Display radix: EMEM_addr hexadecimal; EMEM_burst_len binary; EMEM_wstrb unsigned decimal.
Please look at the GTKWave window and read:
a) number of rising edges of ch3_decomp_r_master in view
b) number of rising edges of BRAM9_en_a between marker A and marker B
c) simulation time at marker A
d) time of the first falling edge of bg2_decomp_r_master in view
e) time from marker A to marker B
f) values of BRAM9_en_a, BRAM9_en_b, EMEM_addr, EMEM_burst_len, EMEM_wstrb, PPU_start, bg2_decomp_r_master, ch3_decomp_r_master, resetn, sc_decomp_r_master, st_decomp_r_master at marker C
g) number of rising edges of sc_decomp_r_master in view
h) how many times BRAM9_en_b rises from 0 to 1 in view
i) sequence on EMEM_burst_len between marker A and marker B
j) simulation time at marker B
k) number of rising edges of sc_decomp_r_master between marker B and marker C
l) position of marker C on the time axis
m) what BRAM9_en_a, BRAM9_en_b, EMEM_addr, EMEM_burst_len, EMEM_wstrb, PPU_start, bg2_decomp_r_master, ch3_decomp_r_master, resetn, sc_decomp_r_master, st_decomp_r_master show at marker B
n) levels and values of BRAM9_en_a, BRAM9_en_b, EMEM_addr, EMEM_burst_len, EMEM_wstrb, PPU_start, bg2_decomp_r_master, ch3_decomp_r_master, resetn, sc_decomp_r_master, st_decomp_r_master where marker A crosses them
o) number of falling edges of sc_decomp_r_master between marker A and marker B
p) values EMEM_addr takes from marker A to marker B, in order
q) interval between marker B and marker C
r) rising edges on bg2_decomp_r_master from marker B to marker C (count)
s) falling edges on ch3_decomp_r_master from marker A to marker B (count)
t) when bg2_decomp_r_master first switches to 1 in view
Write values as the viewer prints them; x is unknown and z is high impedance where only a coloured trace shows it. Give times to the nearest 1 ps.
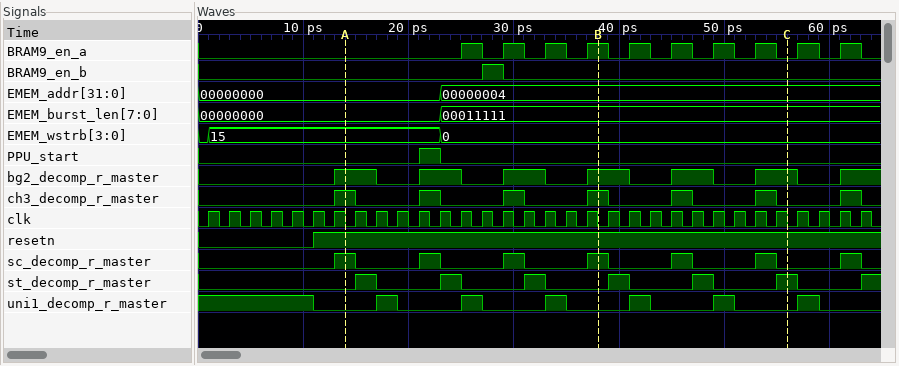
7
4
14 ps
17 ps
24 ps
BRAM9_en_a=0, BRAM9_en_b=0, EMEM_addr=00000004, EMEM_burst_len=00011111, EMEM_wstrb=0, PPU_start=0, bg2_decomp_r_master=1, ch3_decomp_r_master=0, resetn=1, sc_decomp_r_master=0, st_decomp_r_master=1
7
1
00000000, 00011111
38 ps
2
56 ps
BRAM9_en_a=1, BRAM9_en_b=0, EMEM_addr=00000004, EMEM_burst_len=00011111, EMEM_wstrb=0, PPU_start=0, bg2_decomp_r_master=1, ch3_decomp_r_master=1, resetn=1, sc_decomp_r_master=1, st_decomp_r_master=0
BRAM9_en_a=0, BRAM9_en_b=0, EMEM_addr=00000000, EMEM_burst_len=00000000, EMEM_wstrb=15, PPU_start=0, bg2_decomp_r_master=1, ch3_decomp_r_master=1, resetn=1, sc_decomp_r_master=1, st_decomp_r_master=0
3
00000000, 00000004
18 ps
2
3
13 ps
